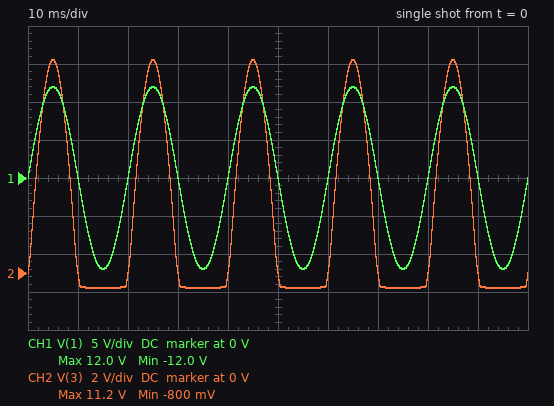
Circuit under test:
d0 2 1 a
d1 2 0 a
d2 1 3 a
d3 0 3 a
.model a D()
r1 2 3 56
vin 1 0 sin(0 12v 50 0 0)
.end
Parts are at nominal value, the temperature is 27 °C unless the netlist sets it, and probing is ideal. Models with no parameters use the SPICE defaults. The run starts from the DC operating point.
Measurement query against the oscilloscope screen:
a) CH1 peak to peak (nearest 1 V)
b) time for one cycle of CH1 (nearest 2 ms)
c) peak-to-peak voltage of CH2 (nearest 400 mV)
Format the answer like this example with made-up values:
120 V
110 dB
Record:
24 V
20 ms
12.0 V
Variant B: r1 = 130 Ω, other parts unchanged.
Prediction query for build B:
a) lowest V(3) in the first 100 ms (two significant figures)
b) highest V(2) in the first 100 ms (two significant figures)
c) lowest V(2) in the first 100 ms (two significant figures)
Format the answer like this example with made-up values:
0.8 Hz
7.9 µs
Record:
-770 mV
770 mV
-11 V
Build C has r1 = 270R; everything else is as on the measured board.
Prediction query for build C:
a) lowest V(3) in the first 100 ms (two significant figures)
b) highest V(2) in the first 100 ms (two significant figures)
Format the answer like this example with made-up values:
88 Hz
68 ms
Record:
-750 mV
750 mV
